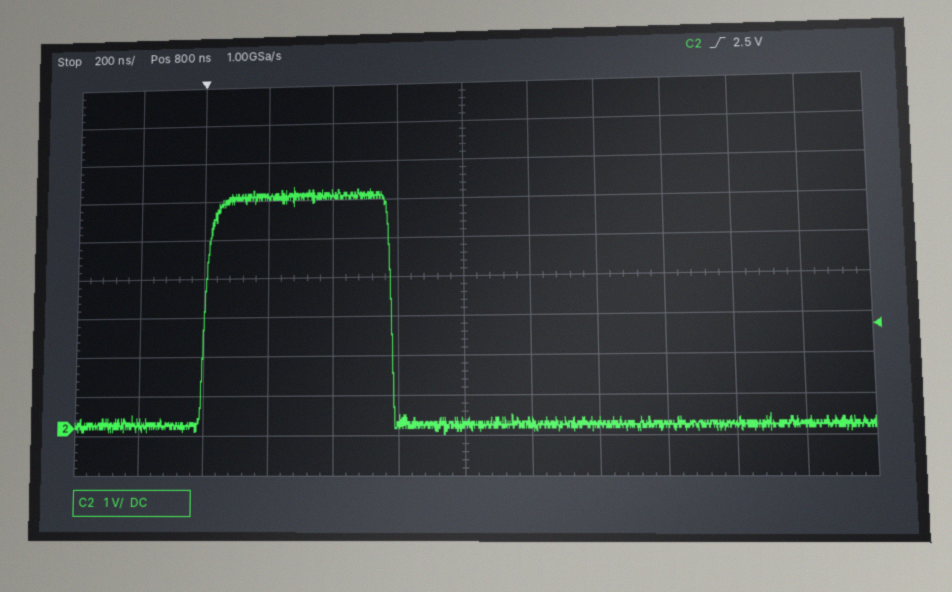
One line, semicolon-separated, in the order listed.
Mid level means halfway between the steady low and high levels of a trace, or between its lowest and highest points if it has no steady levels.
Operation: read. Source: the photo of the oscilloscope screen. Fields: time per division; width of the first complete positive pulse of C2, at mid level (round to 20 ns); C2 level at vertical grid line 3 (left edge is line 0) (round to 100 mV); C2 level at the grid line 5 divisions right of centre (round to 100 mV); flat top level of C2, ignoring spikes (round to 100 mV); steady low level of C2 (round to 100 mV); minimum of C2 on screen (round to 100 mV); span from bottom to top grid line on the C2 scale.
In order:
200 ns; 580 ns; 5.9 V; 100 mV; 5.9 V; 100 mV; -200 mV; 10 V
